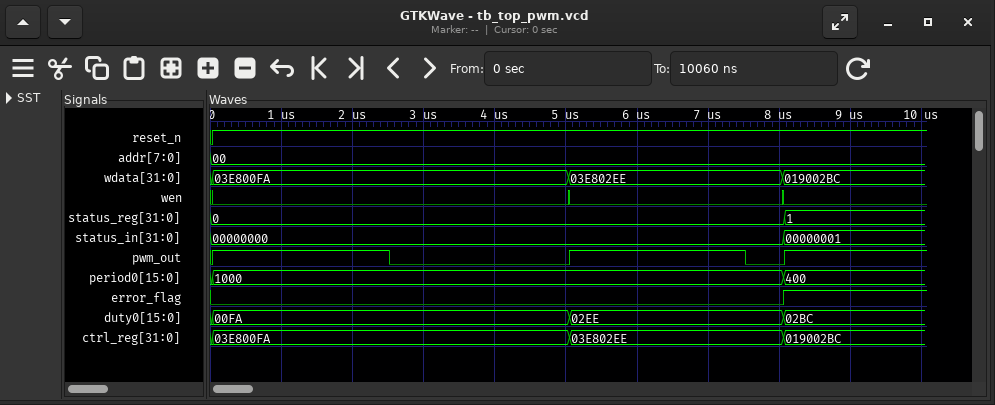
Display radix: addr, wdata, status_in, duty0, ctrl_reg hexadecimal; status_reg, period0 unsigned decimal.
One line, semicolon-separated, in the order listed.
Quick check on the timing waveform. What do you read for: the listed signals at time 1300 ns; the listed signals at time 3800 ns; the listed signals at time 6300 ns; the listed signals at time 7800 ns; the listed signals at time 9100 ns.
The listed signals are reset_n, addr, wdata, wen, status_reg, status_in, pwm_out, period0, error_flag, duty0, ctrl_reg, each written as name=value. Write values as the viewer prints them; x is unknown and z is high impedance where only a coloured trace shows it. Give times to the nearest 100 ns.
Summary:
reset_n=1, addr=00, wdata=03E800FA, wen=0, status_reg=0, status_in=00000000, pwm_out=1, period0=1000, error_flag=0, duty0=00FA, ctrl_reg=03E800FA; reset_n=1, addr=00, wdata=03E800FA, wen=0, status_reg=0, status_in=00000000, pwm_out=0, period0=1000, error_flag=0, duty0=00FA, ctrl_reg=03E800FA; reset_n=1, addr=00, wdata=03E802EE, wen=0, status_reg=0, status_in=00000000, pwm_out=1, period0=1000, error_flag=0, duty0=02EE, ctrl_reg=03E802EE; reset_n=1, addr=00, wdata=03E802EE, wen=0, status_reg=0, status_in=00000000, pwm_out=0, period0=1000, error_flag=0, duty0=02EE, ctrl_reg=03E802EE; reset_n=1, addr=00, wdata=019002BC, wen=0, status_reg=1, status_in=00000001, pwm_out=1, period0=400, error_flag=1, duty0=02BC, ctrl_reg=019002BC
